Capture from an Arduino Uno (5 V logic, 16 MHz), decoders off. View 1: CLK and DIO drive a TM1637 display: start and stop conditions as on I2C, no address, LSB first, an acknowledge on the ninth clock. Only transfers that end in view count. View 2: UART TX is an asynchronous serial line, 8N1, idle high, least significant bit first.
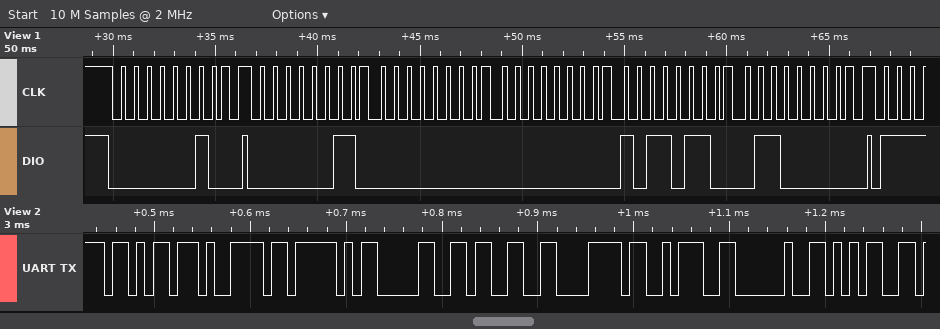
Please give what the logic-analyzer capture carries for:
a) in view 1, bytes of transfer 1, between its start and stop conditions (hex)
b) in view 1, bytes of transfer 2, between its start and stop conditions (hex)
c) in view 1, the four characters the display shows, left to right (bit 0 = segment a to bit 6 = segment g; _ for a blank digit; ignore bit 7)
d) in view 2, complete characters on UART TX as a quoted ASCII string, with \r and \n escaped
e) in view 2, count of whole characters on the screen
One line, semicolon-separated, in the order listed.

40; C0 00 00 6D 06; __51; "ky_03x: 5"; 9
